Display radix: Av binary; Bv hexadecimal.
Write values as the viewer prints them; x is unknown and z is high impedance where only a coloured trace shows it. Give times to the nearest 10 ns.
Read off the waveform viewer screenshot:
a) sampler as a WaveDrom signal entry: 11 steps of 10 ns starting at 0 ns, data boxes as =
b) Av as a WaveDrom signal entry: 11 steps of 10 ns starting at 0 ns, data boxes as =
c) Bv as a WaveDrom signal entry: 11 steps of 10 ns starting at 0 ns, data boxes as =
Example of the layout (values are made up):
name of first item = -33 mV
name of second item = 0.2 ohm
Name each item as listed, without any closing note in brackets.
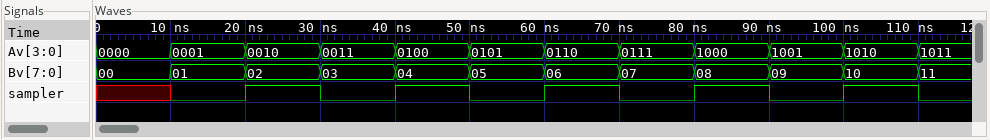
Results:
sampler as a WaveDrom signal entry: 11 steps of 10 ns starting at 0 ns, data boxes as = = {name: 'sampler', wave: 'x0101010101'}
Av as a WaveDrom signal entry: 11 steps of 10 ns starting at 0 ns, data boxes as = = {name: 'Av', wave: '===========', data: '0000 0001 0010 0011 0100 0101 0110 0111 1000 1001 1010'}
Bv as a WaveDrom signal entry: 11 steps of 10 ns starting at 0 ns, data boxes as = = {name: 'Bv', wave: '===========', data: '00 01 02 03 04 05 06 07 08 09 10'}
